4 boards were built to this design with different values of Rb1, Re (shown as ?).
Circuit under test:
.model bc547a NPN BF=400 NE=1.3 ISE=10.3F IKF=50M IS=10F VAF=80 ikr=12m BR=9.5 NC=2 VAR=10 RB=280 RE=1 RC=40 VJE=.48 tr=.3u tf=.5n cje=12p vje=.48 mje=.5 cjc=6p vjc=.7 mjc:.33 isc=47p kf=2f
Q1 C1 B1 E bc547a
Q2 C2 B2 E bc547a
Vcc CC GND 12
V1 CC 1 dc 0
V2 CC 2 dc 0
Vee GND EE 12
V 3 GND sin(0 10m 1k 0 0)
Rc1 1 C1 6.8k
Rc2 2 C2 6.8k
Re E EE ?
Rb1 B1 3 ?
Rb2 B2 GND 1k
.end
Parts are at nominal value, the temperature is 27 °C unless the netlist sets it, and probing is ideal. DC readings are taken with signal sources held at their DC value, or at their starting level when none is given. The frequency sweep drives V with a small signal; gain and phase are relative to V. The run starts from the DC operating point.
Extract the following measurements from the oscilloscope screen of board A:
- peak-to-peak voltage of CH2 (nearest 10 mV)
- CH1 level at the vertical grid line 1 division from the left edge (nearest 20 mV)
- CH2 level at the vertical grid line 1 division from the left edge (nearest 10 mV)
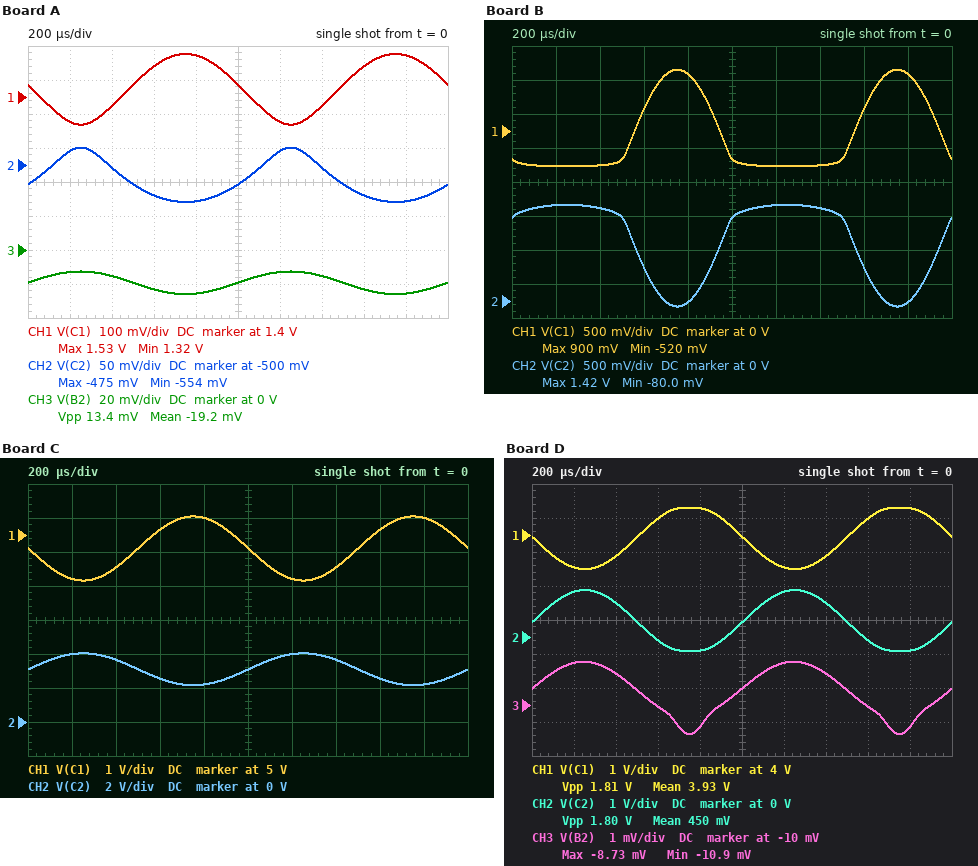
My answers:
80 mV
1.32 V
-480 mV
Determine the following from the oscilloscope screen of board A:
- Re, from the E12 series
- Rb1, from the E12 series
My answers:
3.3 kΩ
3.3 kΩ
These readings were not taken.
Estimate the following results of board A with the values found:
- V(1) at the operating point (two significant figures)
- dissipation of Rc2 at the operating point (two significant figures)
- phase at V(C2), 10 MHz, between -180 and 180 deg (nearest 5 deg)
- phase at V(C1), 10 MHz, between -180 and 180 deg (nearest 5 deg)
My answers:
12 V
23 mW
-25 deg
80 deg
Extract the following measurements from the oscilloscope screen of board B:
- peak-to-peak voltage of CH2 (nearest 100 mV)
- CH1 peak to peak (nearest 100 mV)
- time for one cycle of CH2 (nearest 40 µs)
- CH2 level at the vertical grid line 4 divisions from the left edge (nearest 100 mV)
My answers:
1.5 V
1.4 V
1.00 ms
0 V
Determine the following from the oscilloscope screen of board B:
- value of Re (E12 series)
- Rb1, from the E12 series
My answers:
3.3 kΩ
330 Ω
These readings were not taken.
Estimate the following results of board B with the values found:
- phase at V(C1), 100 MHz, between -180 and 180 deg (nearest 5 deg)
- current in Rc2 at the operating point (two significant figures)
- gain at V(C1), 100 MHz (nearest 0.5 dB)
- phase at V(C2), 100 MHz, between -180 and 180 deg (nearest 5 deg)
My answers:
5 deg
1.6 mA
-5.0 dB
-10 deg
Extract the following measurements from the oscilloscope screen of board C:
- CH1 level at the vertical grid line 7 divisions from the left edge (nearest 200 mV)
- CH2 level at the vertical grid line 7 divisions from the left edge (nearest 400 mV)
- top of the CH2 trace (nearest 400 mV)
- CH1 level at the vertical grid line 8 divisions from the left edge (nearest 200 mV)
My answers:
4.0 V
3.6 V
4.0 V
5.2 V
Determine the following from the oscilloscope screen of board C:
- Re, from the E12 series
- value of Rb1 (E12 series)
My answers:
4.7 kΩ
2.2 kΩ
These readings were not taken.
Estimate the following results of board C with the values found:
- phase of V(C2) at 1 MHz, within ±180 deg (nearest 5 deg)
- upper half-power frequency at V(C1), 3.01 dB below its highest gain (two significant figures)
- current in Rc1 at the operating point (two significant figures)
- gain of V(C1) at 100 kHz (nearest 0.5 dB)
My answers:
-85 deg
130 kHz
1.1 mA
37.5 dB
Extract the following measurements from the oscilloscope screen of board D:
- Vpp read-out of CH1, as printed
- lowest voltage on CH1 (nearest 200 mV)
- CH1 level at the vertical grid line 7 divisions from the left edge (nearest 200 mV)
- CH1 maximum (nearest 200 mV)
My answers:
1.81 V
3.0 V
3.4 V
4.8 V
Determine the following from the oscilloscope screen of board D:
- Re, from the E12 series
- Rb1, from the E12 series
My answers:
3.9 kΩ
3.3 kΩ
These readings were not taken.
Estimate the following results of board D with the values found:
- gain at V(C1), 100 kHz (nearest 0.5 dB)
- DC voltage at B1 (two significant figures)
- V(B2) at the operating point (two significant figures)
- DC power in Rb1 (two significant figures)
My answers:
36.0 dB
-22 mV
-9.5 mV
140 nW
